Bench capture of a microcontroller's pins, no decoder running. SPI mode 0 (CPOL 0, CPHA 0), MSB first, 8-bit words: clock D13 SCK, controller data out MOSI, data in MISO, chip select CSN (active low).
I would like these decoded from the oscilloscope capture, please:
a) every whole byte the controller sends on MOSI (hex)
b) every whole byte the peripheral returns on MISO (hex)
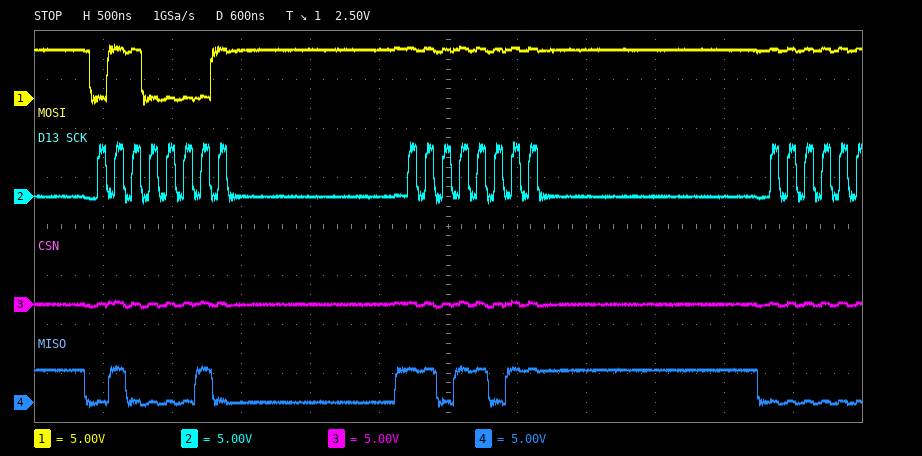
0x61 0xFF
0x42 0xDB
